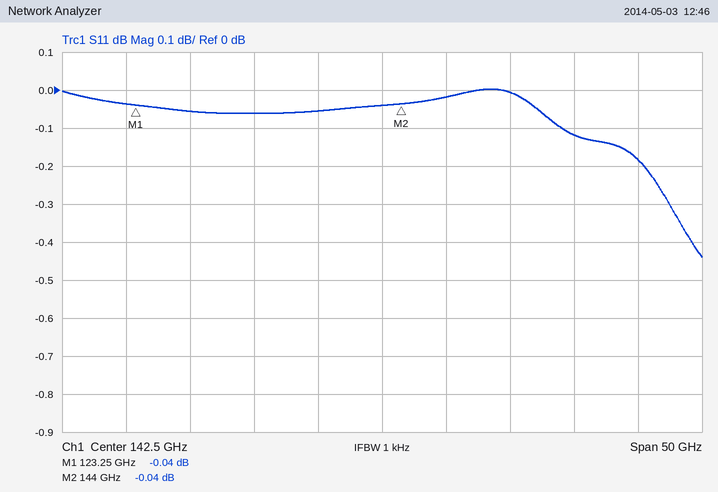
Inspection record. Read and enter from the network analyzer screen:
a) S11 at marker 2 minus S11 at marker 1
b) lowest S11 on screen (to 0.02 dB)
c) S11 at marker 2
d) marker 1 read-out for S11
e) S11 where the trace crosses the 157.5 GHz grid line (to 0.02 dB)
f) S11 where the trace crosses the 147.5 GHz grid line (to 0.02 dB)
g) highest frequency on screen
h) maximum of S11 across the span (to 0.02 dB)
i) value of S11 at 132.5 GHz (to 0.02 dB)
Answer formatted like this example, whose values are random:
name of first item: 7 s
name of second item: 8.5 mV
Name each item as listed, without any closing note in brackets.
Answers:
S11 at marker 2 minus S11 at marker 1: 0.00 dB
lowest S11 on screen: -0.44 dB
S11 at marker 2: -0.04 dB
marker 1 read-out for S11: -0.04 dB
S11 where the trace crosses the 157.5 GHz grid line: -0.12 dB
S11 where the trace crosses the 147.5 GHz grid line: -0.02 dB
highest frequency on screen: 167.5 GHz
maximum of S11 across the span: 0.00 dB
value of S11 at 132.5 GHz: -0.06 dB
